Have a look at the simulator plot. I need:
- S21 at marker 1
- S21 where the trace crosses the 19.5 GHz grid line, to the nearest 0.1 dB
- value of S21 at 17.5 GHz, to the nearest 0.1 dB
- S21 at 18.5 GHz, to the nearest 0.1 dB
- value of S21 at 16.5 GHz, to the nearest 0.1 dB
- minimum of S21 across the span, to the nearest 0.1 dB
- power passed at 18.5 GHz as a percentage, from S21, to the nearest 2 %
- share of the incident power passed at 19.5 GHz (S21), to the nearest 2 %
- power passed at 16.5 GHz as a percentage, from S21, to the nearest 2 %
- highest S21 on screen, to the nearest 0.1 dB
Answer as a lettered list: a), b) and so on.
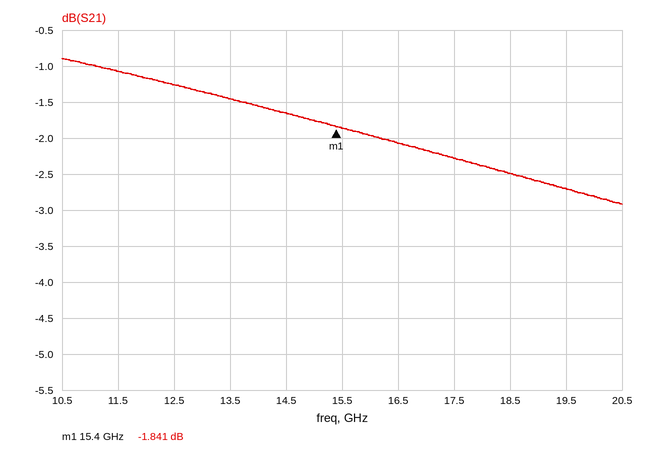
a) -1.841 dB
b) -2.7 dB
c) -2.3 dB
d) -2.5 dB
e) -2.1 dB
f) -2.9 dB
g) 56 %
h) 54 %
i) 62 %
j) -0.9 dB
